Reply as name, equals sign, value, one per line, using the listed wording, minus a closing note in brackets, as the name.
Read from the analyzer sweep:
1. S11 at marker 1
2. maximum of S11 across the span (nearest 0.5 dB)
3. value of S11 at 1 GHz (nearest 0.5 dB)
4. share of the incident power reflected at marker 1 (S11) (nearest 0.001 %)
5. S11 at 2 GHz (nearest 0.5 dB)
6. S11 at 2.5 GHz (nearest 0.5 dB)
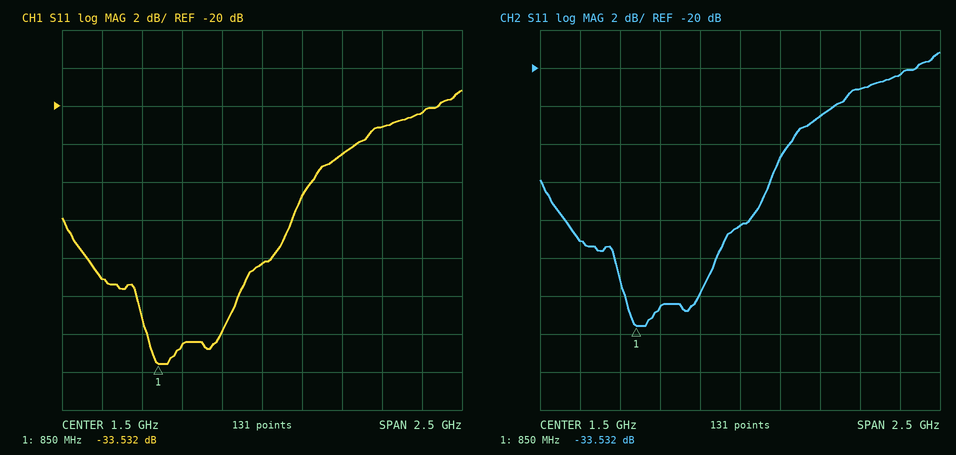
S11 at marker 1 = -33.532 dB
maximum of S11 across the span = -19.0 dB
value of S11 at 1 GHz = -32.5 dB
share of the incident power reflected at marker 1 (S11) = 0.044 %
S11 at 2 GHz = -22.5 dB
S11 at 2.5 GHz = -20.5 dB
